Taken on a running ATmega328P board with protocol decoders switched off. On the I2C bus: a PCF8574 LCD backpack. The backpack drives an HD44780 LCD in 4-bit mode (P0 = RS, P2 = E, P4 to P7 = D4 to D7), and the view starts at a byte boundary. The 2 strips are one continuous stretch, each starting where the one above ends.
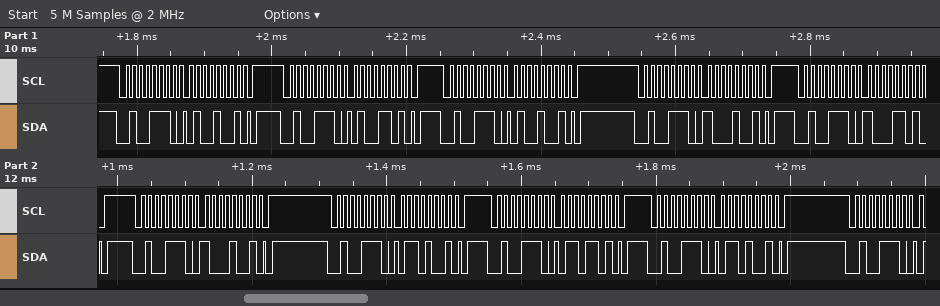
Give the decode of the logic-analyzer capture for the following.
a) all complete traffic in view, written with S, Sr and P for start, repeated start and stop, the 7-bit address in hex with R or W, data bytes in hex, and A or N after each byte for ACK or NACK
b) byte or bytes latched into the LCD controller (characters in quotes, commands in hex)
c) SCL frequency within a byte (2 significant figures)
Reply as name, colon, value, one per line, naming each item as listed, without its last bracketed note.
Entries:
all complete traffic in view, written with S, Sr and P for start, repeated start and stop, the 7-bit address in hex with R or W, data bytes in hex, and A or N after each byte for ACK or NACK: S 27W A 49 A P S 27W A 4D A P S 27W A 49 A P S 27W A 89 A P S 27W A 8D A P S 27W A 89 A P S 27W A 69 A P S 27W A 6D A P S 27W A 69 A P S 27W A
byte or bytes latched into the LCD controller: 'H'
SCL frequency within a byte: 100 kHz
